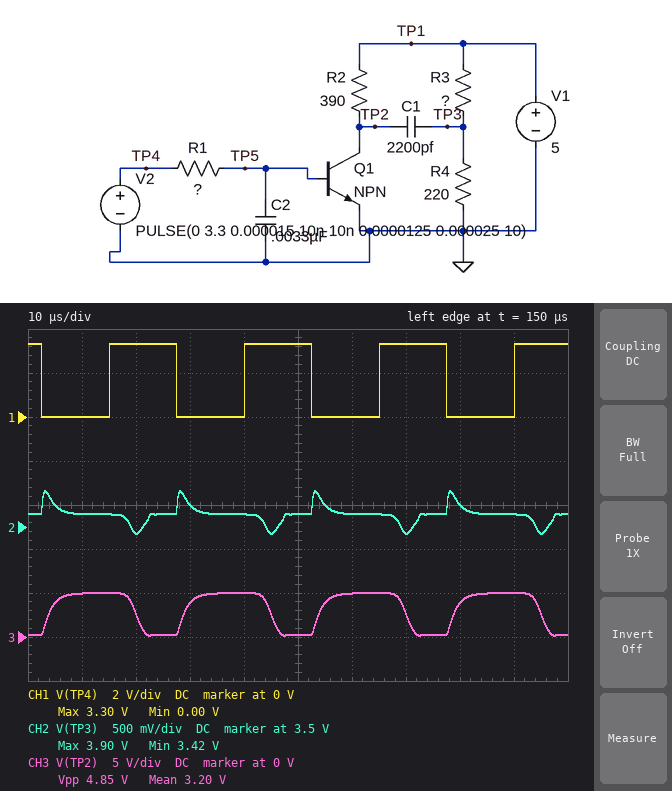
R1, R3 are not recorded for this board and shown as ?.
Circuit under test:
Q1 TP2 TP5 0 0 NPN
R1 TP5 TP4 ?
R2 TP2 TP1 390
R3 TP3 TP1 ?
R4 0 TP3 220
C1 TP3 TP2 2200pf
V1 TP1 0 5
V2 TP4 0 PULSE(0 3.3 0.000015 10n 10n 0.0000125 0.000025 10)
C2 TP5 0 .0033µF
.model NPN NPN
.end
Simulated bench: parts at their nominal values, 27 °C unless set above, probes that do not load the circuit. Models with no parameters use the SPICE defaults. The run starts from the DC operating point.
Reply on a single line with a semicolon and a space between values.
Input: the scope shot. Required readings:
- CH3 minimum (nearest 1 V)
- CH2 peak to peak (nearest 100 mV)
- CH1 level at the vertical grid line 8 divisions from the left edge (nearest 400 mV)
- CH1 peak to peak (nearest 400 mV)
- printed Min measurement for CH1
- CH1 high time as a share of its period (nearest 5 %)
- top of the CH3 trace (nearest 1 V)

0 V; 500 mV; 0 V; 3.2 V; 0.00 V; 50 %; 5 V
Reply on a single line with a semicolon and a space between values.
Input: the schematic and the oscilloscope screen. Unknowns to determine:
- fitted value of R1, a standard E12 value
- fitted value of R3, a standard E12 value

18 kΩ; 82 Ω
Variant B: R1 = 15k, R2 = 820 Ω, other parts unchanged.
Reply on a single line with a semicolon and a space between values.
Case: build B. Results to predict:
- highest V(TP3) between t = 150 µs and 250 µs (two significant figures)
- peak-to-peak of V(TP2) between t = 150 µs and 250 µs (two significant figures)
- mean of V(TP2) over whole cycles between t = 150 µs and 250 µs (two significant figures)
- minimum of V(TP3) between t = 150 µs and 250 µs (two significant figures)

3.8 V; 4.9 V; 2.8 V; 3.2 V
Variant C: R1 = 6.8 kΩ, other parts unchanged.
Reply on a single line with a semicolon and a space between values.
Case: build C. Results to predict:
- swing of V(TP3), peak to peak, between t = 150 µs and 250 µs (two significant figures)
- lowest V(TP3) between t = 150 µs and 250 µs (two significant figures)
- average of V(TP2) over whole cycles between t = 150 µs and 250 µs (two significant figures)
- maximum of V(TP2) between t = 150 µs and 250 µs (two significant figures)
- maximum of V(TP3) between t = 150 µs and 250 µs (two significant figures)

1.3 V; 2.7 V; 2.9 V; 5.0 V; 4.0 V
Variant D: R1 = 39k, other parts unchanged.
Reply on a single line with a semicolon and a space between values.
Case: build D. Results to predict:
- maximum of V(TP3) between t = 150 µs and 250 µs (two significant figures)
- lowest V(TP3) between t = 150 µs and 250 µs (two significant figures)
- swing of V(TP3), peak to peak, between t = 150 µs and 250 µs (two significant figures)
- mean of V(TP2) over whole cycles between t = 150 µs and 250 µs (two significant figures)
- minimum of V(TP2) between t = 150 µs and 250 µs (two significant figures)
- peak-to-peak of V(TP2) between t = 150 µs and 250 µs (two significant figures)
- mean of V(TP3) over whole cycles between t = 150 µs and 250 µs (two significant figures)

3.7 V; 3.6 V; 150 mV; 4.1 V; 2.6 V; 2.4 V; 3.6 V
